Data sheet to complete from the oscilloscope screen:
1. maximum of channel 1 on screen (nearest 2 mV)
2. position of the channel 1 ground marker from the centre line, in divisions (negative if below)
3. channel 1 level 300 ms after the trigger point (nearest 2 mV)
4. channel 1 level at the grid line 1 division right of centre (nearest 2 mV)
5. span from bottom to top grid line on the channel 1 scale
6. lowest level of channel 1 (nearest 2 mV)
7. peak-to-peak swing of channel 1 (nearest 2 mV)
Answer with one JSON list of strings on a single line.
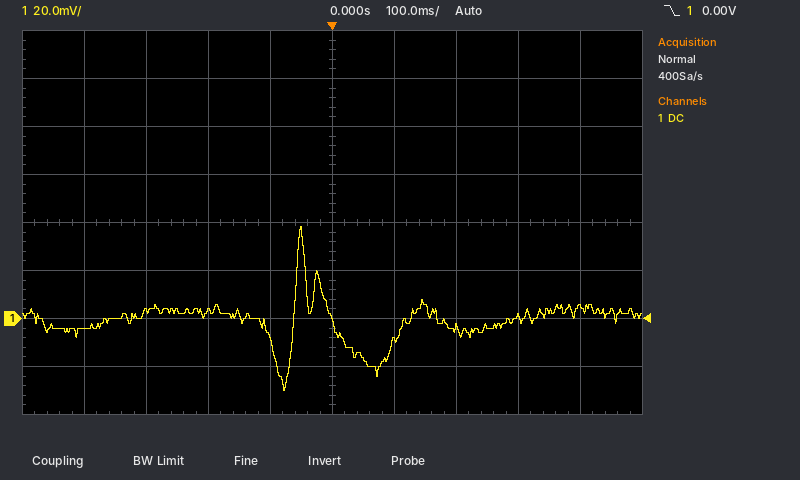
["38 mV", "-2.0 div", "0 mV", "-10 mV", "160 mV", "-30 mV", "68 mV"]
